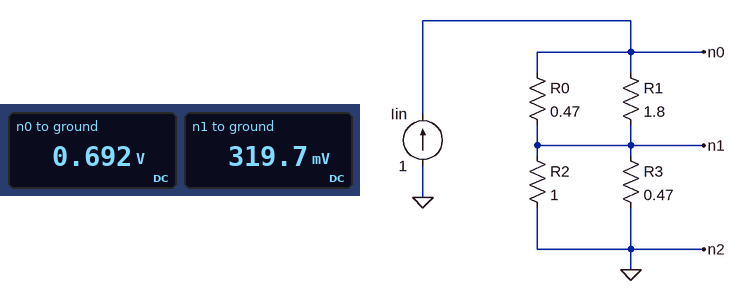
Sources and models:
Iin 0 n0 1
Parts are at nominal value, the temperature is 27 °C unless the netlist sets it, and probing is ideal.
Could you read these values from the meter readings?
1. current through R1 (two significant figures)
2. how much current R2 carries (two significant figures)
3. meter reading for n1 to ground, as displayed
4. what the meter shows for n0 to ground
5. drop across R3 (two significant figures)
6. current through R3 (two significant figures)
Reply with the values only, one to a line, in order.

210 mA
320 mA
319.7 mV
0.692 V
320 mV
680 mA
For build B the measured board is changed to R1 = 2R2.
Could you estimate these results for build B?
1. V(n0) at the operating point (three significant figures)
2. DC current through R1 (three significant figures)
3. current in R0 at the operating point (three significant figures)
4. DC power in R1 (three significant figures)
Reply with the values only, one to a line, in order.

707 mV
176 mA
824 mA
68.2 mW
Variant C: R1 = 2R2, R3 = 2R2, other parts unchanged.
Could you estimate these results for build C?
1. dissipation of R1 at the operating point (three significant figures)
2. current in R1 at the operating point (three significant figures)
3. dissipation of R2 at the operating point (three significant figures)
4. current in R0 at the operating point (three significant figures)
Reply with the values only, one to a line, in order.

68.2 mW
176 mA
473 mW
824 mA
